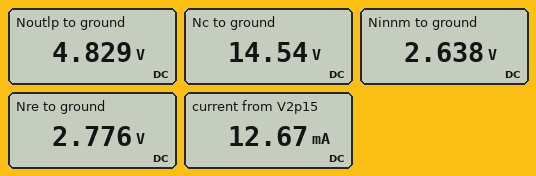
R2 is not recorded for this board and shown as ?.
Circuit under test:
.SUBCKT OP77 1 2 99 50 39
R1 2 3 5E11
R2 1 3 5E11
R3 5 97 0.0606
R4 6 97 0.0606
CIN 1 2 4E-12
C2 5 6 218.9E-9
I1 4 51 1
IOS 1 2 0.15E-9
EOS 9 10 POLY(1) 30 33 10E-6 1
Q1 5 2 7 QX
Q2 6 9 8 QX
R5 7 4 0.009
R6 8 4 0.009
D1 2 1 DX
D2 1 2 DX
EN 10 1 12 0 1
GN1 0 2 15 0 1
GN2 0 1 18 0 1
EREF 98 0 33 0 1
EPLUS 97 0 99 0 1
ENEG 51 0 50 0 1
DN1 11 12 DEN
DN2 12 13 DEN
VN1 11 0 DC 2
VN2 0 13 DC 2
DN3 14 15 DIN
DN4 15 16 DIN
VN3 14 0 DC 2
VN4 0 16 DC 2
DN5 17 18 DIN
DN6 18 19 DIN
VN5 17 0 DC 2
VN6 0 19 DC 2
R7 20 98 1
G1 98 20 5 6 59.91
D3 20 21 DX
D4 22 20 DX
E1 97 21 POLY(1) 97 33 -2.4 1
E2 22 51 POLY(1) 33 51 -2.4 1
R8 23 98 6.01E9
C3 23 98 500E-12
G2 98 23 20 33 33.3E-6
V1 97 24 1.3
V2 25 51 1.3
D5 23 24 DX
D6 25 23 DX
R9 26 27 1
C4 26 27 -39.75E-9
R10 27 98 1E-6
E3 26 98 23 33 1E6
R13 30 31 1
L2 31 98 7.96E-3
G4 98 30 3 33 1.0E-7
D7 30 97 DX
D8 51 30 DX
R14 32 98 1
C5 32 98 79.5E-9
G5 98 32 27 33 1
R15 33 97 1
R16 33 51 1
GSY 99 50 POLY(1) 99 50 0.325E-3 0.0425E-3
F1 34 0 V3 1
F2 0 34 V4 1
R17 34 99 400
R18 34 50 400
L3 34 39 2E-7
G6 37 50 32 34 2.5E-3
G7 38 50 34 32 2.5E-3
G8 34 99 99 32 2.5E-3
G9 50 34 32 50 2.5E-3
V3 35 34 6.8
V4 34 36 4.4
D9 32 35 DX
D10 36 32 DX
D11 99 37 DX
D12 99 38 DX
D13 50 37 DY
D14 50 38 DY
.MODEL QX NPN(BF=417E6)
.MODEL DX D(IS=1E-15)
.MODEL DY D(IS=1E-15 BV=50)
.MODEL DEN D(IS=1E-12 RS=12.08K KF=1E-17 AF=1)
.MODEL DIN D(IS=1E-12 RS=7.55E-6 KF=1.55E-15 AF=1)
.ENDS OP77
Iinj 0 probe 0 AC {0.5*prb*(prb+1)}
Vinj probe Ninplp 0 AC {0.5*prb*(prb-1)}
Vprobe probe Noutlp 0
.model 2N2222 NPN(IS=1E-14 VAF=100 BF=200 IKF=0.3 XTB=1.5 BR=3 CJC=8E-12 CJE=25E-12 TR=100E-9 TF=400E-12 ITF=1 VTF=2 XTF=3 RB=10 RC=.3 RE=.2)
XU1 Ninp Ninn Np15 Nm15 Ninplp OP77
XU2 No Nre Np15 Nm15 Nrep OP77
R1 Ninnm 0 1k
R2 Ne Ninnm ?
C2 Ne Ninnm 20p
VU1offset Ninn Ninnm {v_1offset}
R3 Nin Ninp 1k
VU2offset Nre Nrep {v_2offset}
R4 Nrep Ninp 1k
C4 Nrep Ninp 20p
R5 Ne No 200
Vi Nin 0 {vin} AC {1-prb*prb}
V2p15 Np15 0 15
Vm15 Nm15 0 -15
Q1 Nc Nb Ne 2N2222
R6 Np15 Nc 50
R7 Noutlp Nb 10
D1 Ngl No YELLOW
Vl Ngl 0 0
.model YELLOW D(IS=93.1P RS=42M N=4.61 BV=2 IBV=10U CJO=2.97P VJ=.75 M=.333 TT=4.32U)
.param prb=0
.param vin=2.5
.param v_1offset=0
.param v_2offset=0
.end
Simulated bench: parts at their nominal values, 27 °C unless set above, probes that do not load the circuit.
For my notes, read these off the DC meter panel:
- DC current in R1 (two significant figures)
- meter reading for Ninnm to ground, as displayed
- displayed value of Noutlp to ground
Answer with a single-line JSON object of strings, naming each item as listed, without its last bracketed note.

{"DC current in R1": "2.6 mA", "meter reading for Ninnm to ground, as displayed": "2.638 V", "displayed value of Noutlp to ground": "4.829 V"}
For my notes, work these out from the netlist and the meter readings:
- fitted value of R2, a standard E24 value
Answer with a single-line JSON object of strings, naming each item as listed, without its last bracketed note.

{"fitted value of R2, a standard E24 value": "560 Ω"}
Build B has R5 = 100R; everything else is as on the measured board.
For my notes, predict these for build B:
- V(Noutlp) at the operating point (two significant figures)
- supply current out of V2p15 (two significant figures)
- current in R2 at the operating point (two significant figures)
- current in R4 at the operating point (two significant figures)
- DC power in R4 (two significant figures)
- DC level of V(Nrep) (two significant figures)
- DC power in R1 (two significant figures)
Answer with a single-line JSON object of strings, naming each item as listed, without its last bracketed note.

{"V(Noutlp) at the operating point": "4.9 V", "supply current out of V2p15": "19 mA", "current in R2 at the operating point": "2.7 mA", "current in R4 at the operating point": "180 µA", "DC power in R4": "32 µW", "DC level of V(Nrep)": "2.9 V", "DC power in R1": "7.2 mW"}
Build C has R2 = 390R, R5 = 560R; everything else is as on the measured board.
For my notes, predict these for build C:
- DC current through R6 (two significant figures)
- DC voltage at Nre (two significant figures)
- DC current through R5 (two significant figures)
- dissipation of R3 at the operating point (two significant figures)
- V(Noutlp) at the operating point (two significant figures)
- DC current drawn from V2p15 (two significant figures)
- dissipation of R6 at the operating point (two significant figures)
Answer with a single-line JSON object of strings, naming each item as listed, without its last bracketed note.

{"DC current through R6": "4.2 mA", "DC voltage at Nre": "2.6 V", "DC current through R5": "1.7 mA", "dissipation of R3 at the operating point": "3.1 µW", "V(Noutlp) at the operating point": "4.2 V", "DC current drawn from V2p15": "7.5 mA", "dissipation of R6 at the operating point": "890 µW"}
